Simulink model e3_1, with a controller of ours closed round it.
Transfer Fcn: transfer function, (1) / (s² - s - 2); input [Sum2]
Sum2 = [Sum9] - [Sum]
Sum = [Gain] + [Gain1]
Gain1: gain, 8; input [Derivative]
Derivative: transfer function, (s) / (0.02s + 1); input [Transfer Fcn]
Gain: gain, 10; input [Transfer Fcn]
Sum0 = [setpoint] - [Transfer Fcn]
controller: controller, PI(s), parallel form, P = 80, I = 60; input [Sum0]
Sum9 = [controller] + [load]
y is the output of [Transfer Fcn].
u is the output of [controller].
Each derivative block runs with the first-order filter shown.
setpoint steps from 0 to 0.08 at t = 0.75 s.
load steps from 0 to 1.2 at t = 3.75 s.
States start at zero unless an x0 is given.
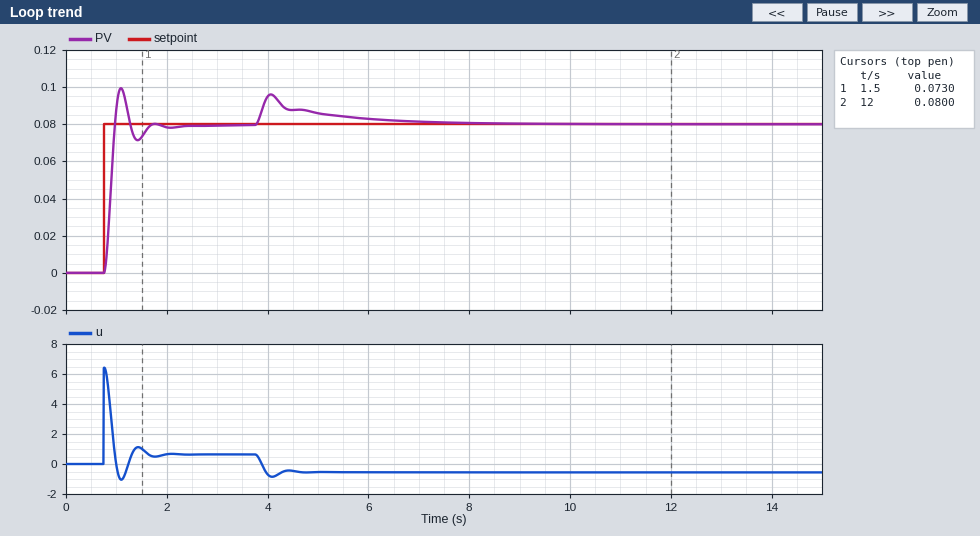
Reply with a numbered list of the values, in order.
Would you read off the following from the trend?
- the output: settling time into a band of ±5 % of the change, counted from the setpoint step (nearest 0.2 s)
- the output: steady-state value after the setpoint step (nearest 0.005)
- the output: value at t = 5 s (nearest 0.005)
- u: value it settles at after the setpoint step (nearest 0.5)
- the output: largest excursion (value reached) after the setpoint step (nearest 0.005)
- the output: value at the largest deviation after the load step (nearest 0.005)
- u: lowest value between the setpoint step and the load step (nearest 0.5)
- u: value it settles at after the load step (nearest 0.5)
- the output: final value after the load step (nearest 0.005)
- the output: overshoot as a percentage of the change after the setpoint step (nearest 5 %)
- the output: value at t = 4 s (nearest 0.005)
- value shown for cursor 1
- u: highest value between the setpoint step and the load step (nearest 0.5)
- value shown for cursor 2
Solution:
1. 0.8 s
2. 0.080
3. 0.085
4. 0.5
5. 0.100
6. 0.095
7. -1.0
8. -0.5
9. 0.080
10. 25 %
11. 0.095
12. 0.0730
13. 6.5
14. 0.0800
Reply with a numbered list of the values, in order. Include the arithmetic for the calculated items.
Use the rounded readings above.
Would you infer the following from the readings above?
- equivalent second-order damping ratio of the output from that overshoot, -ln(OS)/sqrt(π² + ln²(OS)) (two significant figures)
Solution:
1. ln(0.25) = -1.386; 1.386 / sqrt(9.870 + 1.922) = 0.40
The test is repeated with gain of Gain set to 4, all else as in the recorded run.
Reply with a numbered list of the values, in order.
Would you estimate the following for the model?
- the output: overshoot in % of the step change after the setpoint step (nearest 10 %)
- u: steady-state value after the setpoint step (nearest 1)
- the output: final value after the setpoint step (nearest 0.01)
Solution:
1. 30 %
2. 0
3. 0.08
